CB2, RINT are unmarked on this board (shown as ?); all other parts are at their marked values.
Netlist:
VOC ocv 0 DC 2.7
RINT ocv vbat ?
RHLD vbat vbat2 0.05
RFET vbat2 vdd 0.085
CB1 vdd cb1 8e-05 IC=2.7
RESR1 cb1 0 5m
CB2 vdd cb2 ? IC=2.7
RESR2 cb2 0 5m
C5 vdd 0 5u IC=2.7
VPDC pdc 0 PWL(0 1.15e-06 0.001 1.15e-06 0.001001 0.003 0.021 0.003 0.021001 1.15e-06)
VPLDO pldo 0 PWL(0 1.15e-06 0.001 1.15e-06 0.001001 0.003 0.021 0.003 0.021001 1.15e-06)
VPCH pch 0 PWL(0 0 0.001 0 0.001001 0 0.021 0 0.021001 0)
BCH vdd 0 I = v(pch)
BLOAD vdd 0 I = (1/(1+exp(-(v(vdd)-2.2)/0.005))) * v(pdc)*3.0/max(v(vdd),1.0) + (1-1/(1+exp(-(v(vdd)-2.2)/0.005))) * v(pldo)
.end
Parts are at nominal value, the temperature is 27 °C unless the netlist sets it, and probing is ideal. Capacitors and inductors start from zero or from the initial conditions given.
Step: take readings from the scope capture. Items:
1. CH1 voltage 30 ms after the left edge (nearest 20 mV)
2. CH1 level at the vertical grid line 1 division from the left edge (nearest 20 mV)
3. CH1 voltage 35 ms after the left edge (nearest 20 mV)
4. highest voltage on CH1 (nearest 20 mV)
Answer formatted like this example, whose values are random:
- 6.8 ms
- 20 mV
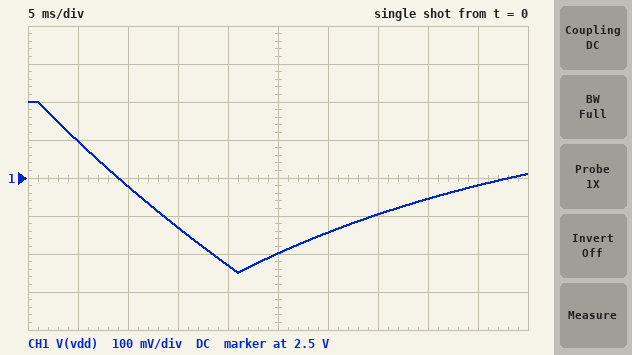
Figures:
- 2.36 V
- 2.60 V
- 2.40 V
- 2.70 V
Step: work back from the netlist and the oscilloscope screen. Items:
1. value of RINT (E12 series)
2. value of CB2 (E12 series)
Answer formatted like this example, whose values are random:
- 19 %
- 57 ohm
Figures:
- 270 Ω
- 39 µF
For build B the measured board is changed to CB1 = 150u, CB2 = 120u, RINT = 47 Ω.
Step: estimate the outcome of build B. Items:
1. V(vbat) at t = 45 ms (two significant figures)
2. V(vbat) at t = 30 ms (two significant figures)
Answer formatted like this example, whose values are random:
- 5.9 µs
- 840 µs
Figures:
- 2.7 V
- 2.6 V
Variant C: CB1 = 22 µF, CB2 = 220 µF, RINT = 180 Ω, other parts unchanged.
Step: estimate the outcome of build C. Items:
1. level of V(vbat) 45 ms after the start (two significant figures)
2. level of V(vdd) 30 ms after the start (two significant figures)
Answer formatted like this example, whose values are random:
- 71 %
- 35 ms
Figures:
- 2.6 V
- 2.5 V
